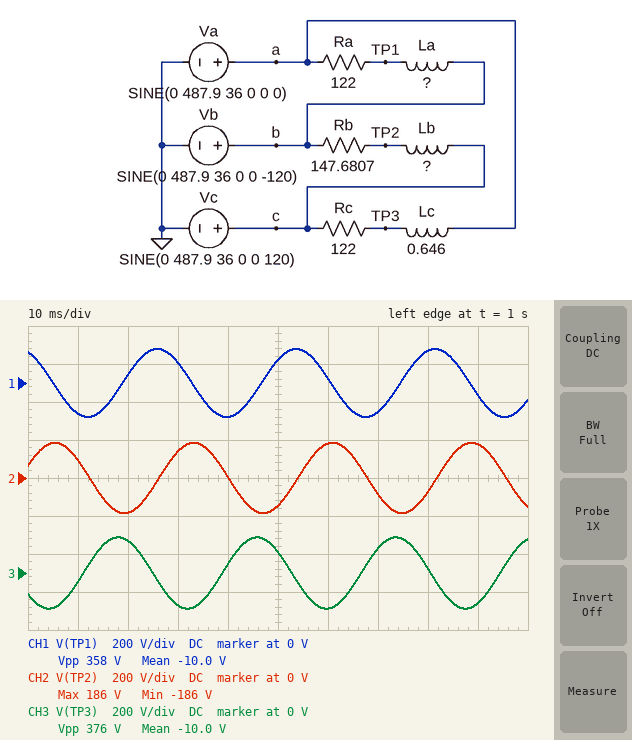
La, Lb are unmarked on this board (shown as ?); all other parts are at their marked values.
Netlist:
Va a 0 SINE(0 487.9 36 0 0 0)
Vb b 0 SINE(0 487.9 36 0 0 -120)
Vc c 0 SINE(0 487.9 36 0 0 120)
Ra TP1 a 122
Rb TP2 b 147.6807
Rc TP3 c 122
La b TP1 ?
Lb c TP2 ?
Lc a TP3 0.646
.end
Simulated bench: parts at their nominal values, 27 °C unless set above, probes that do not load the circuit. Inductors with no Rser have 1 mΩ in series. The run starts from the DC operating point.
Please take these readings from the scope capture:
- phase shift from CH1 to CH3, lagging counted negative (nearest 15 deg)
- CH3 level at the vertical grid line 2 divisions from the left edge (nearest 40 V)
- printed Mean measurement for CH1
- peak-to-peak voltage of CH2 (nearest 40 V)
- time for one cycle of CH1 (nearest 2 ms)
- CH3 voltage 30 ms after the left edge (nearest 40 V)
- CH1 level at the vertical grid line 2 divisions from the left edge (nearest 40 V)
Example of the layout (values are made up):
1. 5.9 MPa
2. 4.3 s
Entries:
1. 105 deg
2. 160 V
3. -10.0 V
4. 360 V
5. 28 ms
6. -160 V
7. 40 V
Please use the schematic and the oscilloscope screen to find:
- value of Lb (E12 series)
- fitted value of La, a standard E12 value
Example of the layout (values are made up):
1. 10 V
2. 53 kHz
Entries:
1. 560 mH
2. 560 mH
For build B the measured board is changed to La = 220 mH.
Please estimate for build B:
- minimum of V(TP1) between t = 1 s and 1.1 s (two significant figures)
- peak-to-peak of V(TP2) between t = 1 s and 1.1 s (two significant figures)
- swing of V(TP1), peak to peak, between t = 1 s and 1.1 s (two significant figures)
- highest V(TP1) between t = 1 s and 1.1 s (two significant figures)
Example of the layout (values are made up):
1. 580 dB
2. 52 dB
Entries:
1. -310 V
2. 370 V
3. 610 V
4. 310 V
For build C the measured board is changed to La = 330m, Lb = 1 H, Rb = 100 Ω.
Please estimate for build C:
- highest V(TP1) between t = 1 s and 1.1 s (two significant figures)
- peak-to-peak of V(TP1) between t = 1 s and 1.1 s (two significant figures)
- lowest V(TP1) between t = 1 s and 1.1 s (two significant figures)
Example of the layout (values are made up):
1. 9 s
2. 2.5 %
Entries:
1. 230 V
2. 470 V
3. -230 V
